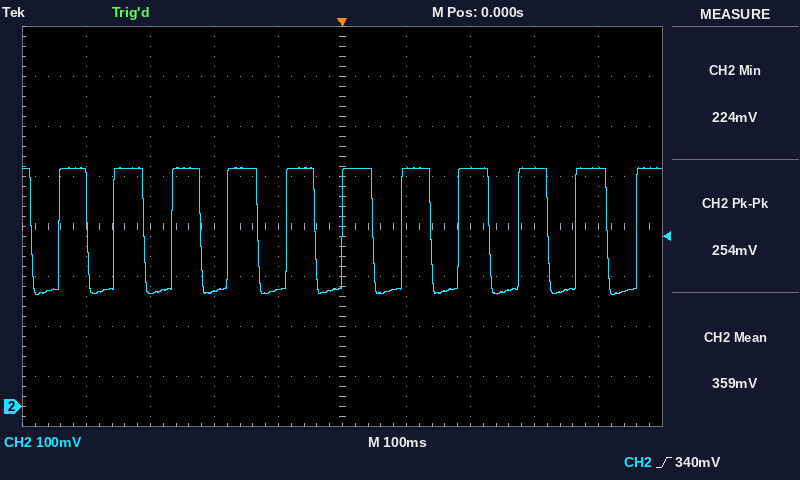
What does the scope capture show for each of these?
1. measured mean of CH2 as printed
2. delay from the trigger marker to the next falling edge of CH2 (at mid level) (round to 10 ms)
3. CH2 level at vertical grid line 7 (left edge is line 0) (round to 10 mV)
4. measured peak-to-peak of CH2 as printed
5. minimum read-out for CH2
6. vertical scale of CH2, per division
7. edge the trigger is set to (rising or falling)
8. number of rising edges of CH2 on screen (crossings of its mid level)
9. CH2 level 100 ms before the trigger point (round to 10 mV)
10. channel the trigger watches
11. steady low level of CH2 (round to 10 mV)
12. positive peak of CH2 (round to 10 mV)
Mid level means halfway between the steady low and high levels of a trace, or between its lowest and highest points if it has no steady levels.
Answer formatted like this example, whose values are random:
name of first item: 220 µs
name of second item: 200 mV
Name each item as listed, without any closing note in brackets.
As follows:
measured mean of CH2 as printed: 359 mV
delay from the trigger marker to the next falling edge of CH2 (at mid level): 50 ms
CH2 level at vertical grid line 7 (left edge is line 0): 480 mV
measured peak-to-peak of CH2 as printed: 254 mV
minimum read-out for CH2: 224 mV
vertical scale of CH2, per division: 100 mV
edge the trigger is set to: rising
number of rising edges of CH2 on screen: 11
CH2 level 100 ms before the trigger point: 230 mV
channel the trigger watches: CH2
steady low level of CH2: 230 mV
positive peak of CH2: 480 mV
